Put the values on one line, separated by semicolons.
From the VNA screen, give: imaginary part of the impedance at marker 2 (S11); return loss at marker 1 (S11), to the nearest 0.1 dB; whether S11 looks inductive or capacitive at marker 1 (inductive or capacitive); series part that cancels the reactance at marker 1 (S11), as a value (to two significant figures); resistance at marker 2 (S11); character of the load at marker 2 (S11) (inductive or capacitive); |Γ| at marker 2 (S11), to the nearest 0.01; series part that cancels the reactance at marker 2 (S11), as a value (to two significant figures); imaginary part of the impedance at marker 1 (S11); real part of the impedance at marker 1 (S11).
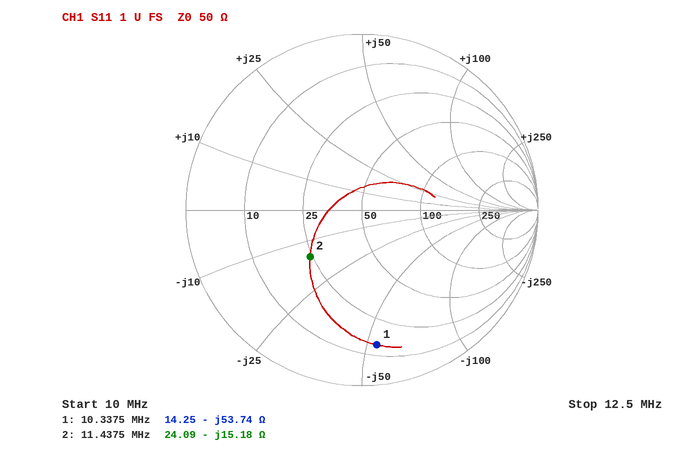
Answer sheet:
-15.18 Ω; 2.3 dB; capacitive; 830 nH; 24.09 Ω; capacitive; 0.40; 210 nH; -53.74 Ω; 14.25 Ω
